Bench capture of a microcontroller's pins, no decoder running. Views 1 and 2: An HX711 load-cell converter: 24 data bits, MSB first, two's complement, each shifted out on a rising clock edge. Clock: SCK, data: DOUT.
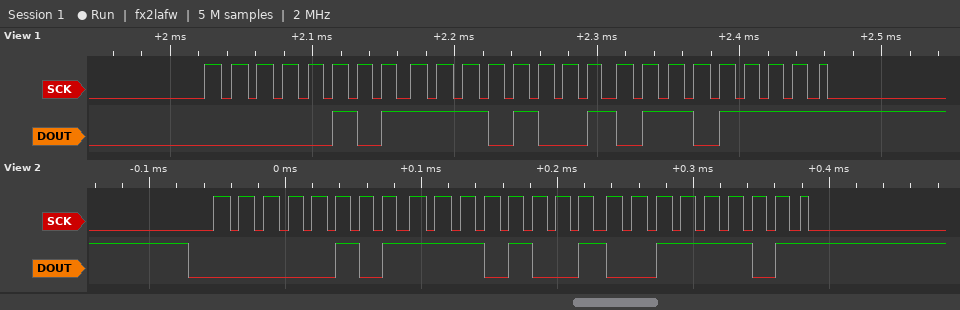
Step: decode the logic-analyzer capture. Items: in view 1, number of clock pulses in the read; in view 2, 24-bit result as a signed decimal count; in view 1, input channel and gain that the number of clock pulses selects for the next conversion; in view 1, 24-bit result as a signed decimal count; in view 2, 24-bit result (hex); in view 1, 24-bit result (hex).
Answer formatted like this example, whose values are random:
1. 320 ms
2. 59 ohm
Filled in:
1. 25
2. 387389
3. channel A, gain 128
4. 387439
5. 0x05E93D
6. 0x05E96F
